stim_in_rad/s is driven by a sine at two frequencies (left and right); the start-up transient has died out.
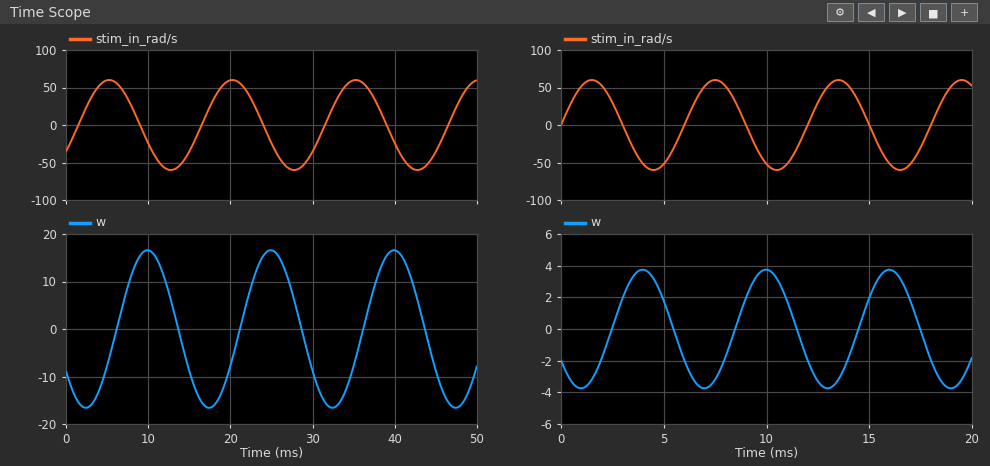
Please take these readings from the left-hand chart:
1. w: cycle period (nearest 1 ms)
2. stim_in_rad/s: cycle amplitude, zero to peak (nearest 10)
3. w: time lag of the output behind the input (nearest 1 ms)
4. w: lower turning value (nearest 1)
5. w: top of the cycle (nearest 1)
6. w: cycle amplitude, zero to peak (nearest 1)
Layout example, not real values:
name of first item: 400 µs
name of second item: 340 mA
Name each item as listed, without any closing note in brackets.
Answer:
w: cycle period: 15 ms
stim_in_rad/s: cycle amplitude, zero to peak: 60
w: time lag of the output behind the input: 5 ms
w: lower turning value: -17
w: top of the cycle: 17
w: cycle amplitude, zero to peak: 17
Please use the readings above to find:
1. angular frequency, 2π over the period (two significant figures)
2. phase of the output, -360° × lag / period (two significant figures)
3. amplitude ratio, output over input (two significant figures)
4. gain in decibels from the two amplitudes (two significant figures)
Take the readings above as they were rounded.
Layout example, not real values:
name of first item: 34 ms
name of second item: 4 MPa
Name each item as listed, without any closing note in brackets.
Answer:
angular frequency, 2π over the period: 0.42 rad/ms
phase of the output, -360° × lag / period: -120°
amplitude ratio, output over input: 0.28
gain in decibels from the two amplitudes: -11 dB
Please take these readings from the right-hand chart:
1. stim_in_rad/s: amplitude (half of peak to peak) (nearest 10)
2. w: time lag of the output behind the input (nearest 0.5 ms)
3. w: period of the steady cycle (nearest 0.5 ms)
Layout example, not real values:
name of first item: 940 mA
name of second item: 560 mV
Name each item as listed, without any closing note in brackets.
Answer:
stim_in_rad/s: amplitude (half of peak to peak): 60
w: time lag of the output behind the input: 2.5 ms
w: period of the steady cycle: 6.0 ms
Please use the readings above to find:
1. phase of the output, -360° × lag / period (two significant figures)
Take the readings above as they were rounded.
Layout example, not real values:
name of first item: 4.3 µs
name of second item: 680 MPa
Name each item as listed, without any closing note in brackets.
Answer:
phase of the output, -360° × lag / period: -150°
